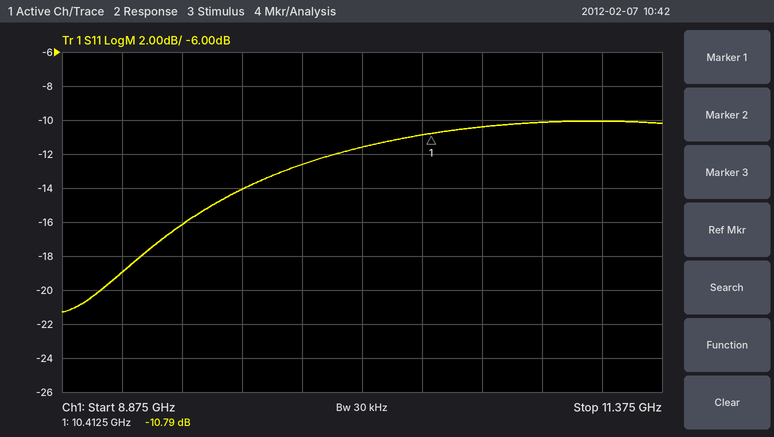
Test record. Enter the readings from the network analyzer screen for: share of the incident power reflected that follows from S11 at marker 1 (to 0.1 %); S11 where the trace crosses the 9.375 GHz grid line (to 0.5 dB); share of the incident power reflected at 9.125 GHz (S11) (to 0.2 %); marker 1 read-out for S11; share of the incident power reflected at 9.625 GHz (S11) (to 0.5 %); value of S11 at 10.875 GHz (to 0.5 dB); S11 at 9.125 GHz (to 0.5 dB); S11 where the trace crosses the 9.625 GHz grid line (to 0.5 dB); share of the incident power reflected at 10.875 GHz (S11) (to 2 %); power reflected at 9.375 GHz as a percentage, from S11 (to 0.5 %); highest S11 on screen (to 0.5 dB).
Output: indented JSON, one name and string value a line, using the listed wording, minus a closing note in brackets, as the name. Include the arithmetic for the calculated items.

{
  "share of the incident power reflected that follows from S11 at marker 1": "10^(-10.79/10) ≈ 8.3 %",
  "S11 where the trace crosses the 9.375 GHz grid line": "-16.0 dB",
  "share of the incident power reflected at 9.125 GHz (S11)": "10^(-19/10) ≈ 1.26 %, so 1.2 % to the nearest 0.2 %",
  "marker 1 read-out for S11": "-10.79 dB",
  "share of the incident power reflected at 9.625 GHz (S11)": "10^(-14/10) ≈ 4.0 %",
  "value of S11 at 10.875 GHz": "-10.0 dB",
  "S11 at 9.125 GHz": "-19.0 dB",
  "S11 where the trace crosses the 9.625 GHz grid line": "-14.0 dB",
  "share of the incident power reflected at 10.875 GHz (S11)": "10^(-10/10) ≈ 10 %",
  "power reflected at 9.375 GHz as a percentage, from S11": "10^(-16/10) ≈ 2.5 %",
  "highest S11 on screen": "-10.0 dB"
}
